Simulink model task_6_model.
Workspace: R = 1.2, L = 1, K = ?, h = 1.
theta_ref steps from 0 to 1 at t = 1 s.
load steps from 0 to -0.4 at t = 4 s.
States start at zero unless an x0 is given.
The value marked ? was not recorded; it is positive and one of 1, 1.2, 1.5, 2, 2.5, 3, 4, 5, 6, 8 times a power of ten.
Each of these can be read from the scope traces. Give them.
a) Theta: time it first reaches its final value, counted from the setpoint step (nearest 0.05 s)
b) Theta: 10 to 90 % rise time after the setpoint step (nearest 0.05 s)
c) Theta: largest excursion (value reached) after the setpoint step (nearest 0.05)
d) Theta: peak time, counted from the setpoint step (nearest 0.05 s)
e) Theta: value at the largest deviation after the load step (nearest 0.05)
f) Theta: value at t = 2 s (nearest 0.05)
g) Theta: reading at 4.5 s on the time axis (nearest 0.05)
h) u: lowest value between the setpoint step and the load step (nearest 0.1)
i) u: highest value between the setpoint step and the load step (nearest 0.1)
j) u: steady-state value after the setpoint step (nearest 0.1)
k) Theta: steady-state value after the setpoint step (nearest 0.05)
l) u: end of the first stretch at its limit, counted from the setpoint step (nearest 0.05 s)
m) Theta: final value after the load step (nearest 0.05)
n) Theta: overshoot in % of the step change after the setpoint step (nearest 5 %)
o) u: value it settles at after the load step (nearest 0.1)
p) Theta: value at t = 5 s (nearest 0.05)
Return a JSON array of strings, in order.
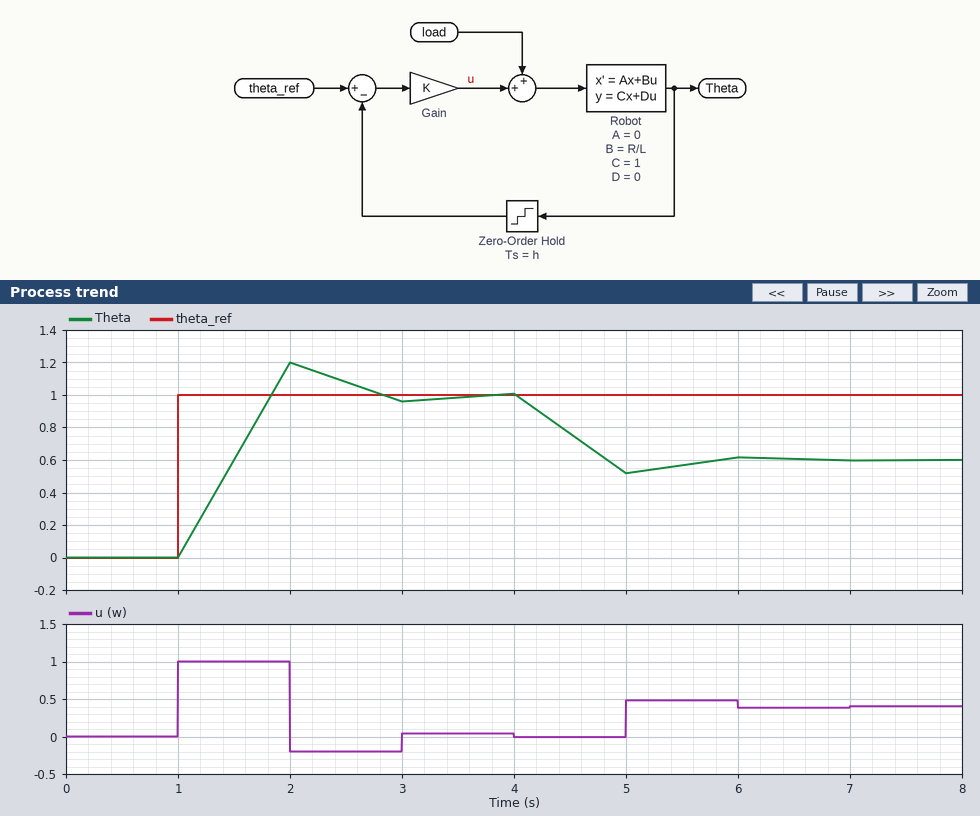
["0.85 s", "0.65 s", "1.20", "1.00 s", "0.50", "1.20", "0.75", "-0.2", "1.0", "0.0", "1.00", "1.00 s", "0.60", "20 %", "0.4", "0.50"]
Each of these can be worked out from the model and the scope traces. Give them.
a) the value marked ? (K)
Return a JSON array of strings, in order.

["1"]
